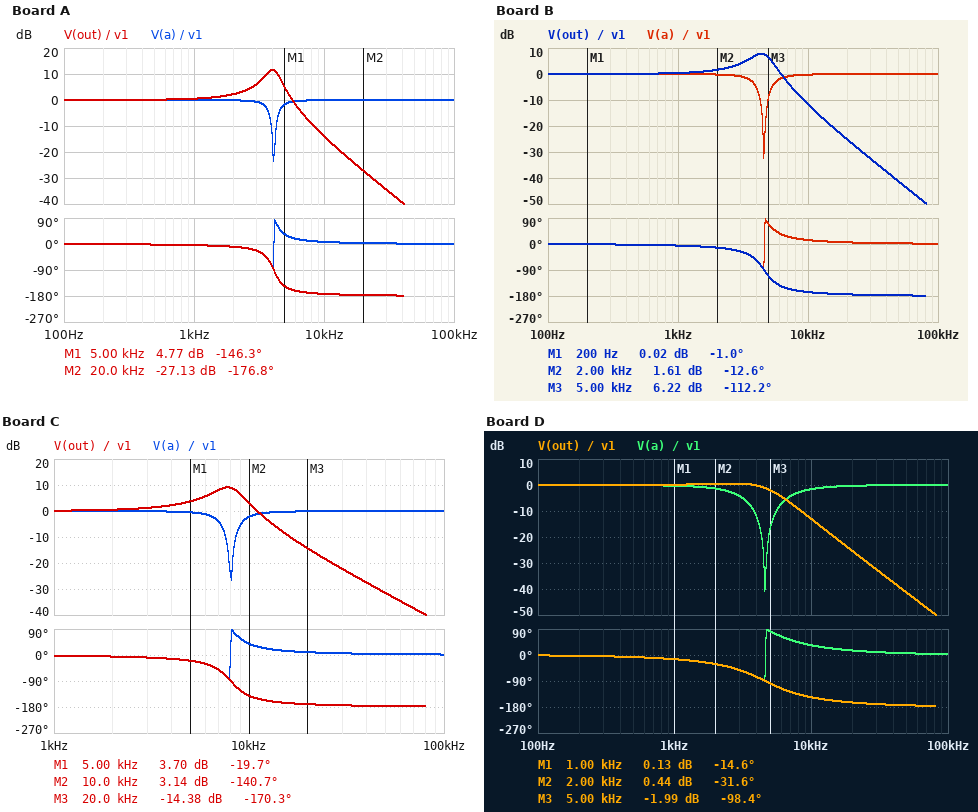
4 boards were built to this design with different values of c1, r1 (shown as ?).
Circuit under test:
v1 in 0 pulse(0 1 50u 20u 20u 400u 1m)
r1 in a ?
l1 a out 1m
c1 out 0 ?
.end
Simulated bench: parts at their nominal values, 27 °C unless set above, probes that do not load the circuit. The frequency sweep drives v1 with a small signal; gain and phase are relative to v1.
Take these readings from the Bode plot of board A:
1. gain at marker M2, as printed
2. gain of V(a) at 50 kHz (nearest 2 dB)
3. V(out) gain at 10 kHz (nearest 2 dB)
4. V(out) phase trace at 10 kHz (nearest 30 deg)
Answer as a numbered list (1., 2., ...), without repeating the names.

1. -27.13 dB
2. 0 dB
3. -14 dB
4. -180 deg
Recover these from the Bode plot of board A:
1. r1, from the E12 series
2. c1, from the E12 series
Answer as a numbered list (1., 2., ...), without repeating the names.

1. 6.8 Ω
2. 1.5 µF
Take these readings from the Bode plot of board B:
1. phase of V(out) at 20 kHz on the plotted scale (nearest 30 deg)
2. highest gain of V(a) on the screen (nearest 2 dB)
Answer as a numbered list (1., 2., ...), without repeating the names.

1. -180 deg
2. 0 dB
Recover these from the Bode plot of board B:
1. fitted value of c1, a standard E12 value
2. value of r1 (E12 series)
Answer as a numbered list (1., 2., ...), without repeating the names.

1. 1.2 µF
2. 12 Ω
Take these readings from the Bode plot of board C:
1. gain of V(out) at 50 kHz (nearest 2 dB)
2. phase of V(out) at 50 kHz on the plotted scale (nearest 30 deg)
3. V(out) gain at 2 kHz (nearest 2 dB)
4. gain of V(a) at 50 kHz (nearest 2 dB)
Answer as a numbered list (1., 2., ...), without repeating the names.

1. -32 dB
2. -180 deg
3. 0 dB
4. 0 dB
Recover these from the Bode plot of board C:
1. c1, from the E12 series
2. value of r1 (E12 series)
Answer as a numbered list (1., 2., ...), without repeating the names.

1. 390 nF
2. 18 Ω
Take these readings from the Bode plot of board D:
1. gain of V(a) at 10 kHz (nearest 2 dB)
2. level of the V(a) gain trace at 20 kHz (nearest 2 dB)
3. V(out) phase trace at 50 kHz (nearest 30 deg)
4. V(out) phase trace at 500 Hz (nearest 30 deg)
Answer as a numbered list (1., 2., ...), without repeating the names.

1. -2 dB
2. 0 dB
3. -180 deg
4. 0 deg
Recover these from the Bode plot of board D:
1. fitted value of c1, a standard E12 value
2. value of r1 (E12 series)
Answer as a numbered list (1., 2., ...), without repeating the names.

1. 1.2 µF
2. 33 Ω
